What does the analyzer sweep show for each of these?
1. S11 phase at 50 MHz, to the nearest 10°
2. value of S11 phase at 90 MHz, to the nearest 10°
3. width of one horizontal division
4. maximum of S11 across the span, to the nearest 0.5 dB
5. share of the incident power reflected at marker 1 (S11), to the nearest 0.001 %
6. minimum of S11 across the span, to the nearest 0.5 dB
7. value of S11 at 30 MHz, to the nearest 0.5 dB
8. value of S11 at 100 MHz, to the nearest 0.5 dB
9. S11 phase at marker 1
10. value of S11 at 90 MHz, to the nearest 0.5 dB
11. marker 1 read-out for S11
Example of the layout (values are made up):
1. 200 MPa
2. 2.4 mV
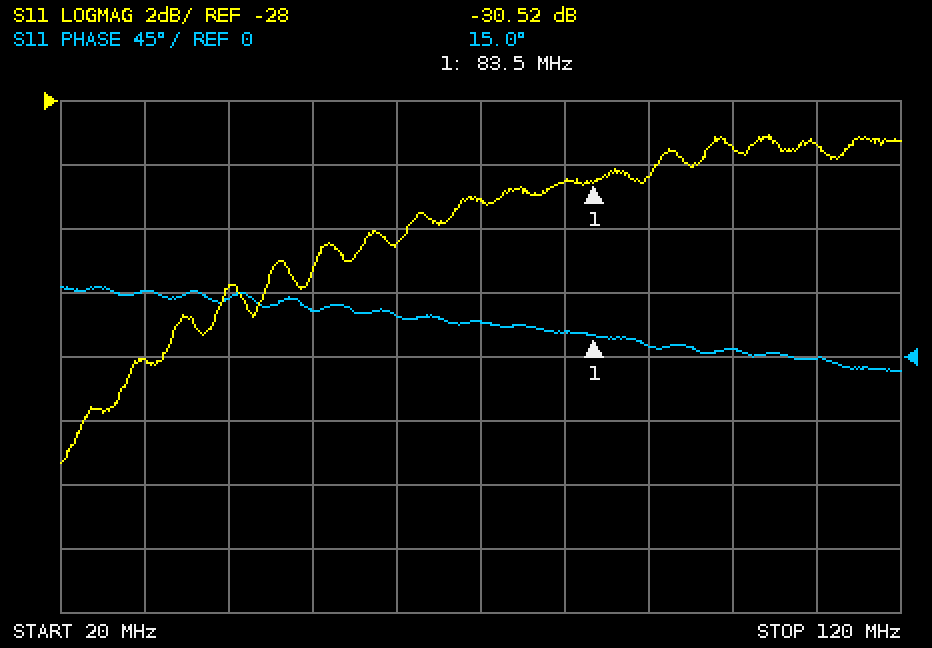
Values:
1. 30°
2. 10°
3. 10 MHz
4. -29.0 dB
5. 0.089 %
6. -39.5 dB
7. -36.0 dB
8. -29.5 dB
9. 15.0°
10. -30.5 dB
11. -30.52 dB
